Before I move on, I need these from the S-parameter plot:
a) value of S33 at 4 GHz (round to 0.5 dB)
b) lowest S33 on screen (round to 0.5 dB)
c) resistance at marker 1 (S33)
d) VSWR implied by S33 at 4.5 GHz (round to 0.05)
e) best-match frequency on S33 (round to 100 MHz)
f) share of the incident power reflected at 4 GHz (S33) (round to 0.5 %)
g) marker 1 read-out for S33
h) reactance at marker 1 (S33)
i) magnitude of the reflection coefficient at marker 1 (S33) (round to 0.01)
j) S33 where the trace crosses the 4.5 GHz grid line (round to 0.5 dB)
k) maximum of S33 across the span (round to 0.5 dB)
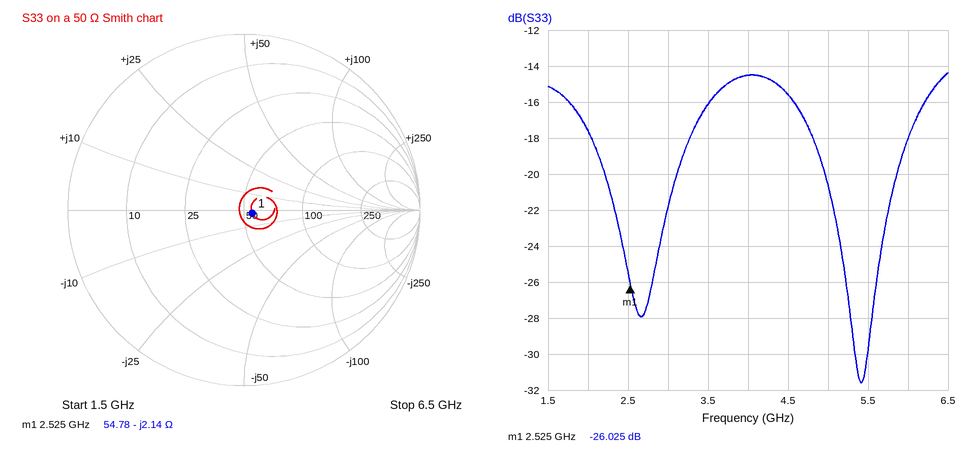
-14.5 dB
-31.5 dB
54.78 Ω
1.40
5.4 GHz
3.5 %
-26.025 dB
-2.14 Ω
0.05
-15.5 dB
-14.5 dB
